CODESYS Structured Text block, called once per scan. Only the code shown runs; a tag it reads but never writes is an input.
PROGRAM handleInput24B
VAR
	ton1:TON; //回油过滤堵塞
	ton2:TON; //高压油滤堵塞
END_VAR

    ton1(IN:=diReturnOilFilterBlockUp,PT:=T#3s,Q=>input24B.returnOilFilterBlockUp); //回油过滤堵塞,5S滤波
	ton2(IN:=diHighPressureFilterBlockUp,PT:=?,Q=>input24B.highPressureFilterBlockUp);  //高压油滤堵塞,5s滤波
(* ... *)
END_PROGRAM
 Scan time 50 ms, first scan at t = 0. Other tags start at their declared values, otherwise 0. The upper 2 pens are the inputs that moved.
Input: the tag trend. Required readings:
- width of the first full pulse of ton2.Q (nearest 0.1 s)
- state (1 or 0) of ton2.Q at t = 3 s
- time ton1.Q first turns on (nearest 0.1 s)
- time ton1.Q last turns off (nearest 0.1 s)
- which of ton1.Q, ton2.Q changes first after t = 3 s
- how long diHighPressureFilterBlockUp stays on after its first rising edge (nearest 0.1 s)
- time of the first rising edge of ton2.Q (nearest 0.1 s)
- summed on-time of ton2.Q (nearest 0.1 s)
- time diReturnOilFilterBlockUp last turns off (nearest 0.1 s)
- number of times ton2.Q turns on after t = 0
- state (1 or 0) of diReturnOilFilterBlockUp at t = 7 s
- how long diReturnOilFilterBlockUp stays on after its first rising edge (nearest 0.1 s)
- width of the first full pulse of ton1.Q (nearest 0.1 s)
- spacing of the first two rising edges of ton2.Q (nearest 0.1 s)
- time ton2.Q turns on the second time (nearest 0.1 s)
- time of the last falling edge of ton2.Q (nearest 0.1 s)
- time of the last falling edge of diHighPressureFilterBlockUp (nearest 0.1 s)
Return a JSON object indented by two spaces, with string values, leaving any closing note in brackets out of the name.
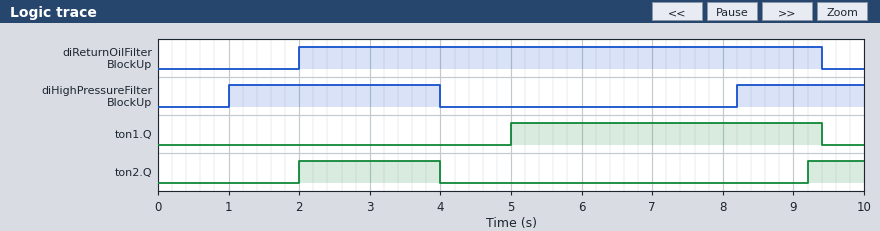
{
  "width of the first full pulse of ton2.Q": "2.0 s",
  "state (1 or 0) of ton2.Q at t = 3 s": "1",
  "time ton1.Q first turns on": "5.0 s",
  "time ton1.Q last turns off": "9.4 s",
  "which of ton1.Q, ton2.Q changes first after t = 3 s": "ton2.Q",
  "how long diHighPressureFilterBlockUp stays on after its first rising edge": "3.0 s",
  "time of the first rising edge of ton2.Q": "2.0 s",
  "summed on-time of ton2.Q": "2.8 s",
  "time diReturnOilFilterBlockUp last turns off": "9.4 s",
  "number of times ton2.Q turns on after t = 0": "2",
  "state (1 or 0) of diReturnOilFilterBlockUp at t = 7 s": "1",
  "how long diReturnOilFilterBlockUp stays on after its first rising edge": "7.4 s",
  "width of the first full pulse of ton1.Q": "4.4 s",
  "spacing of the first two rising edges of ton2.Q": "7.2 s",
  "time ton2.Q turns on the second time": "9.2 s",
  "time of the last falling edge of ton2.Q": "4.0 s",
  "time of the last falling edge of diHighPressureFilterBlockUp": "4.0 s"
}
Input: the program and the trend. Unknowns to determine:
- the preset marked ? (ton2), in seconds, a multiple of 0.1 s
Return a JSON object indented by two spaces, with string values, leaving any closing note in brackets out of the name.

{
  "the preset marked ? (ton2), in seconds, a multiple of 0.1 s": "1.0 s"
}
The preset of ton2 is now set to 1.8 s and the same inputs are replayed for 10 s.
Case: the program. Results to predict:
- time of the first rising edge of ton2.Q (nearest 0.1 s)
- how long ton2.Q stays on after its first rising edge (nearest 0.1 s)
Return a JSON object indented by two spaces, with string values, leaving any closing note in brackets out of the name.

{
  "time of the first rising edge of ton2.Q": "2.8 s",
  "how long ton2.Q stays on after its first rising edge": "1.2 s"
}
